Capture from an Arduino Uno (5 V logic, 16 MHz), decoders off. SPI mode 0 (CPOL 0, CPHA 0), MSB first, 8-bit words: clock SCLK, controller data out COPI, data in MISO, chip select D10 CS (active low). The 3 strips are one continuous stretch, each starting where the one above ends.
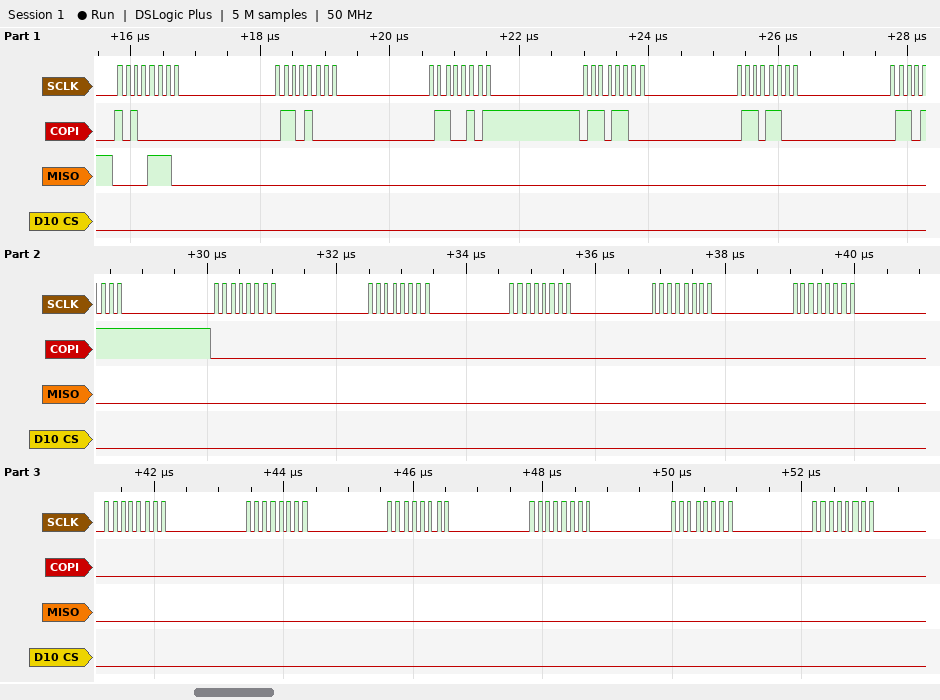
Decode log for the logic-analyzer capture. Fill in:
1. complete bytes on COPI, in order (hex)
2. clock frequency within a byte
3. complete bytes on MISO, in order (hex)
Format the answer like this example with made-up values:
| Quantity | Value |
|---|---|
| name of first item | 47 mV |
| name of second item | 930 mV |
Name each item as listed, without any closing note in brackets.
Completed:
| Quantity | Value |
|---|---|
| complete bytes on COPI, in order | A0 68 65 6C 6C 6F 00 00 00 00 00 00 00 00 00 00 00 |
| clock frequency within a byte | 8 MHz |
| complete bytes on MISO, in order | 0E 00 00 00 00 00 00 00 00 00 00 00 00 00 00 00 00 |
